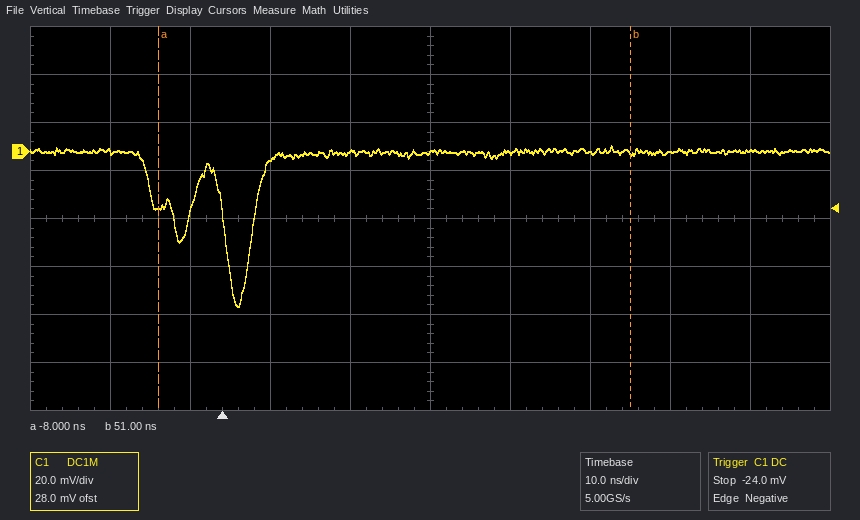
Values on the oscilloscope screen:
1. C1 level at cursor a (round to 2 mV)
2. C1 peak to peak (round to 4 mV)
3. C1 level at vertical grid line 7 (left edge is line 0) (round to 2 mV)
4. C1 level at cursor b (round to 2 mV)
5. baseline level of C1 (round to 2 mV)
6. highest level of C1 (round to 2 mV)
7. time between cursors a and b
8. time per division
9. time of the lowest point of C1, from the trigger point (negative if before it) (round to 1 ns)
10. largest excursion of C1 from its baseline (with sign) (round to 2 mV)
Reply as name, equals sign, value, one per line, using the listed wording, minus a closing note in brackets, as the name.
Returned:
C1 level at cursor a = -24 mV
C1 peak to peak = 68 mV
C1 level at vertical grid line 7 (left edge is line 0) = 0 mV
C1 level at cursor b = 0 mV
baseline level of C1 = 0 mV
highest level of C1 = 2 mV
time between cursors a and b = 59 ns
time per division = 10 ns
time of the lowest point of C1, from the trigger point (negative if before it) = +2 ns
largest excursion of C1 from its baseline (with sign) = -64 mV
